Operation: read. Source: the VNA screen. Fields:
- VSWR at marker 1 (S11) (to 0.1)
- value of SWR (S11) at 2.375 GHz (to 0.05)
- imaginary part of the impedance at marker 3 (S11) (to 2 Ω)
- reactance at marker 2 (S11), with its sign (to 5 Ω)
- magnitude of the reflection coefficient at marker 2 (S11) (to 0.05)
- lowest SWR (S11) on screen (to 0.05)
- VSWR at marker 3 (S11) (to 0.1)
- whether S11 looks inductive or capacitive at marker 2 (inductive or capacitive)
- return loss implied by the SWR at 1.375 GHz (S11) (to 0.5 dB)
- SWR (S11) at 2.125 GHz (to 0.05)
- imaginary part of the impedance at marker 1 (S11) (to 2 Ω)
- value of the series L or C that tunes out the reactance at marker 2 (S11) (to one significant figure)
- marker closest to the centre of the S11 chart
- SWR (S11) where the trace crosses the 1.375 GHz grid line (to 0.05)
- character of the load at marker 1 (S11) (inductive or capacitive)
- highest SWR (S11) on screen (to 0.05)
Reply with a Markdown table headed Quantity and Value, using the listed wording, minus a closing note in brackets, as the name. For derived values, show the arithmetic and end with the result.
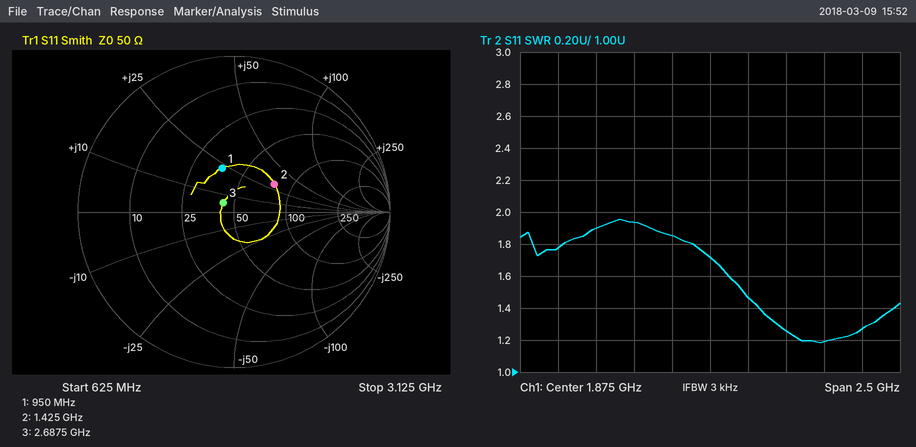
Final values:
| Quantity | Value |
|---|---|
| VSWR at marker 1 (S11) | 1.8 |
| value of SWR (S11) at 2.375 GHz | 1.25 |
| imaginary part of the impedance at marker 3 (S11) | +6 Ω |
| reactance at marker 2 (S11), with its sign | +30 Ω |
| magnitude of the reflection coefficient at marker 2 (S11) | 0.30 |
| lowest SWR (S11) on screen | 1.20 |
| VSWR at marker 3 (S11) | 1.2 |
| whether S11 looks inductive or capacitive at marker 2 | inductive |
| return loss implied by the SWR at 1.375 GHz (S11) | −20 log10((1.95 − 1)/(1.95 + 1)) ≈ 9.84 dB, so 10.0 dB to the nearest 0.5 dB |
| SWR (S11) at 2.125 GHz | 1.45 |
| imaginary part of the impedance at marker 1 (S11) | +22 Ω |
| value of the series L or C that tunes out the reactance at marker 2 (S11) | C = 1/(2π × 1.425 GHz × 30 Ω) ≈ 4 pF |
| marker closest to the centre of the S11 chart | marker 3 |
| SWR (S11) where the trace crosses the 1.375 GHz grid line | 1.95 |
| character of the load at marker 1 (S11) | inductive |
| highest SWR (S11) on screen | 1.95 |
